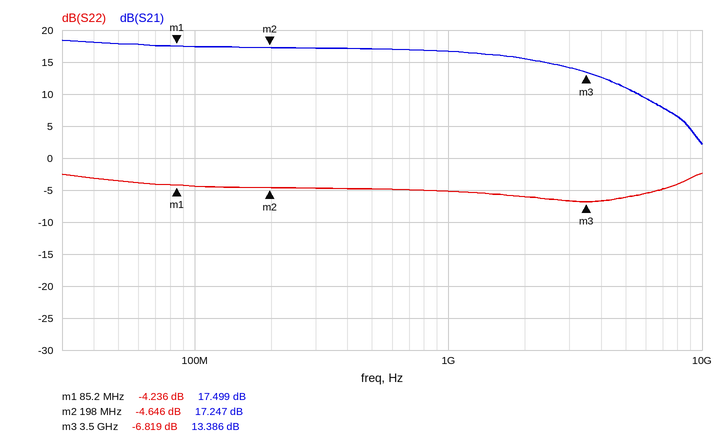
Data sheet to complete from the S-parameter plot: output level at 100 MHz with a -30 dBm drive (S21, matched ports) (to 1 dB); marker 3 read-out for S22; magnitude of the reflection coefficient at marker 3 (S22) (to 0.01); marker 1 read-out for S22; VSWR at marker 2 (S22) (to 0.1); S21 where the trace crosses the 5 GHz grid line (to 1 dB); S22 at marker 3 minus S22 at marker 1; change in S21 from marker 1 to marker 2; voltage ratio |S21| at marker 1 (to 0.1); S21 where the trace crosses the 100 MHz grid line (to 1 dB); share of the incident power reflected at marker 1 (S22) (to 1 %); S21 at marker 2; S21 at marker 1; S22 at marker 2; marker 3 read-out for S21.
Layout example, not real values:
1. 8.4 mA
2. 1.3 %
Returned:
1. -13 dBm
2. -6.819 dB
3. 0.46
4. -4.236 dB
5. 3.8
6. 11 dB
7. -2.583 dB
8. -0.252 dB
9. 7.5
10. 17 dB
11. 38 %
12. 17.247 dB
13. 17.499 dB
14. -4.646 dB
15. 13.386 dB
